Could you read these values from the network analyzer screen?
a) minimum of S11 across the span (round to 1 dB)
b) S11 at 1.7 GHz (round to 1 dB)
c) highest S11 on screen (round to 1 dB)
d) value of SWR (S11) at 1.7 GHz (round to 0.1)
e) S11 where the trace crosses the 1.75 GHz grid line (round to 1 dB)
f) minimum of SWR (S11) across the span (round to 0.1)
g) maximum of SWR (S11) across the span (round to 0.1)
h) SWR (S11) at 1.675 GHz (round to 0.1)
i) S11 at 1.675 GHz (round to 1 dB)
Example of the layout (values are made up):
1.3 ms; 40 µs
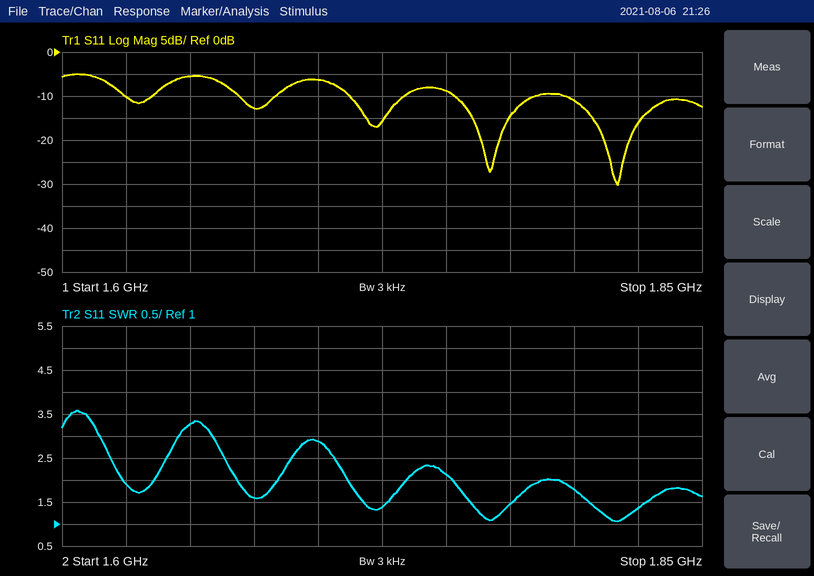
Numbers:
-30 dB; -6 dB; -5 dB; 2.9; -9 dB; 1.1; 3.6; 1.6; -13 dB
